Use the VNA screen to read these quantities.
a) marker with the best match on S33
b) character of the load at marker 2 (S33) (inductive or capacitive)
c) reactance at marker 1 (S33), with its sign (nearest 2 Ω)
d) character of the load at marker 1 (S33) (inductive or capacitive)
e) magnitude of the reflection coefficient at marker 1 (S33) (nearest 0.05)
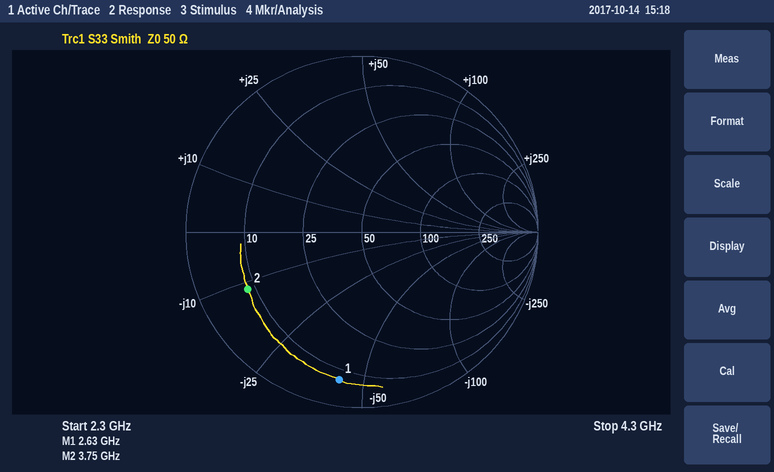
marker 2
capacitive
-42 Ω
capacitive
0.85
